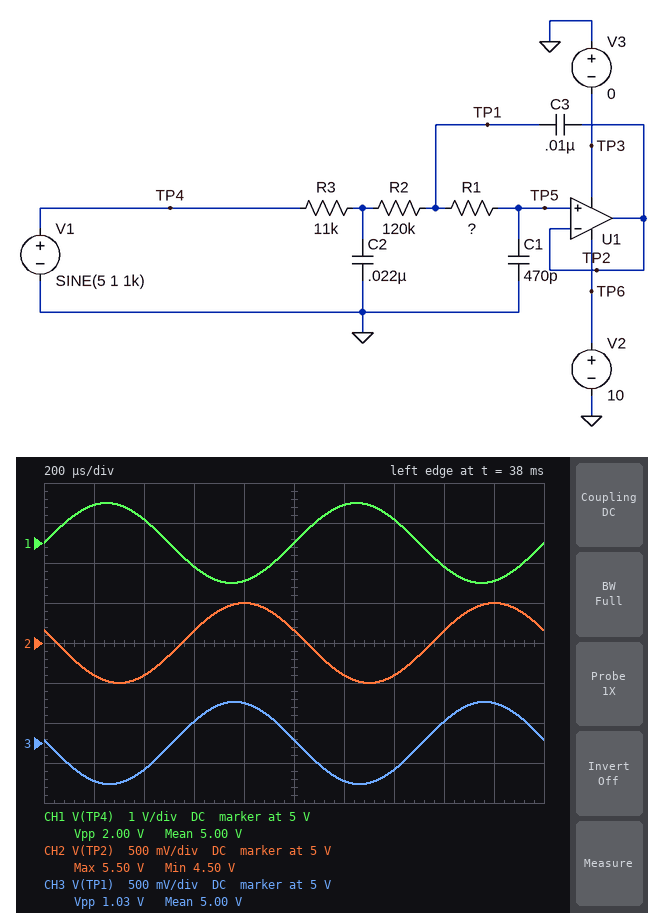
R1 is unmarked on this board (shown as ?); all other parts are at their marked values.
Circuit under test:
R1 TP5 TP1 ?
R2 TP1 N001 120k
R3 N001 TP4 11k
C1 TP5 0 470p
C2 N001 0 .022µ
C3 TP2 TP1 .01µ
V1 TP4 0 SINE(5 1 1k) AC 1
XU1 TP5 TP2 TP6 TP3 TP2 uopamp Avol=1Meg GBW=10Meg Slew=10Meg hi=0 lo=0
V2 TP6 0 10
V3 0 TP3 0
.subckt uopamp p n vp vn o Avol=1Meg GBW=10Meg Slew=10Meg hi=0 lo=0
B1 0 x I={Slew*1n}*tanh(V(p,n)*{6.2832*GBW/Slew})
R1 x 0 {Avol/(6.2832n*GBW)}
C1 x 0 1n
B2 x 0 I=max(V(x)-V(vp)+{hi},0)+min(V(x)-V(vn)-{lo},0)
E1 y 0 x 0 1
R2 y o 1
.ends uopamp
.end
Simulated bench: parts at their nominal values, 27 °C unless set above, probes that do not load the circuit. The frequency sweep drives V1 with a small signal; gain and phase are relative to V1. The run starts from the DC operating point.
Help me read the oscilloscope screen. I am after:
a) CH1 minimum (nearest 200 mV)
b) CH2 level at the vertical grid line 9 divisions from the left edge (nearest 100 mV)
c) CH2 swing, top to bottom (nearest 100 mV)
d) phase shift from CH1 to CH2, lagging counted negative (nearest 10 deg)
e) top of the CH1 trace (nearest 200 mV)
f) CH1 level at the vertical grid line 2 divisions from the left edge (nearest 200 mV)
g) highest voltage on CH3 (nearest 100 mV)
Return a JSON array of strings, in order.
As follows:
["4.0 V", "5.5 V", "1.0 V", "160 deg", "6.0 V", "5.6 V", "5.5 V"]
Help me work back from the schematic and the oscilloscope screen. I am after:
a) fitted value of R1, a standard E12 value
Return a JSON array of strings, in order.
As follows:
["82 kΩ"]
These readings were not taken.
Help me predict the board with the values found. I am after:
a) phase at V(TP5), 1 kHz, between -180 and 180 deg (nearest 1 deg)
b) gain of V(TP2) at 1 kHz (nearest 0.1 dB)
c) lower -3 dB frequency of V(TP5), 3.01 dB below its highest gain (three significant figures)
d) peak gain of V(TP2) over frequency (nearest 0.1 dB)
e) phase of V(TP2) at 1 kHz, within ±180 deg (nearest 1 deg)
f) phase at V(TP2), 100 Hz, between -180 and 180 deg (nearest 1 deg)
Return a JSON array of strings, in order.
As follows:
["162 deg", "-6.0 dB", "259 Hz", "3.4 dB", "162 deg", "-12 deg"]
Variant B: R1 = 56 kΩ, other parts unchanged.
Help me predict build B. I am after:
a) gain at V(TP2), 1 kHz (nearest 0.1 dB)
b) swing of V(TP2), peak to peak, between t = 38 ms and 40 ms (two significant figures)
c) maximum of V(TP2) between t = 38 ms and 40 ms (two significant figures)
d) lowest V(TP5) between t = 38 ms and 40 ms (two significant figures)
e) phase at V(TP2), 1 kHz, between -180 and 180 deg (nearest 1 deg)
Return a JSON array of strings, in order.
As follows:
["-1.3 dB", "1.7 V", "5.9 V", "4.1 V", "-171 deg"]
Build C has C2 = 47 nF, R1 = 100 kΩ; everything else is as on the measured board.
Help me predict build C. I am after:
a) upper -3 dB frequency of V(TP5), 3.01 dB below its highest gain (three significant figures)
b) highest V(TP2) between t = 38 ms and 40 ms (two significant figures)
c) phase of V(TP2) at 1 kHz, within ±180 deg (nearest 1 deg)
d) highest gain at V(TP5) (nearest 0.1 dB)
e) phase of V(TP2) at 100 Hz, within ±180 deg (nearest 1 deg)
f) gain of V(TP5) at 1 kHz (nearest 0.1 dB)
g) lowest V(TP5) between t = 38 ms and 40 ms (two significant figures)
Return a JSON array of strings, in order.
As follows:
["729 Hz", "5.2 V", "137 deg", "0 dB", "-22 deg", "-13.7 dB", "4.8 V"]
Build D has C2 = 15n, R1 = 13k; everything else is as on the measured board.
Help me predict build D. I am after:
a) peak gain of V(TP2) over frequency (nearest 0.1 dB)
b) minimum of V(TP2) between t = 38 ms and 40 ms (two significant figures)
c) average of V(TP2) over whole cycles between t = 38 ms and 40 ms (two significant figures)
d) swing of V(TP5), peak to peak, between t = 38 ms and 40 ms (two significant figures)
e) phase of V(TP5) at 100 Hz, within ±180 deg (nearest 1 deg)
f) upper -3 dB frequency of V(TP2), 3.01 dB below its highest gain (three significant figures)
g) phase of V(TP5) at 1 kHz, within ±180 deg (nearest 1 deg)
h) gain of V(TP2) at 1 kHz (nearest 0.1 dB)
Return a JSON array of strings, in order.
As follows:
["0 dB", "4.2 V", "5.0 V", "1.7 V", "-8 deg", "1.62 kHz", "-77 deg", "-1.5 dB"]
